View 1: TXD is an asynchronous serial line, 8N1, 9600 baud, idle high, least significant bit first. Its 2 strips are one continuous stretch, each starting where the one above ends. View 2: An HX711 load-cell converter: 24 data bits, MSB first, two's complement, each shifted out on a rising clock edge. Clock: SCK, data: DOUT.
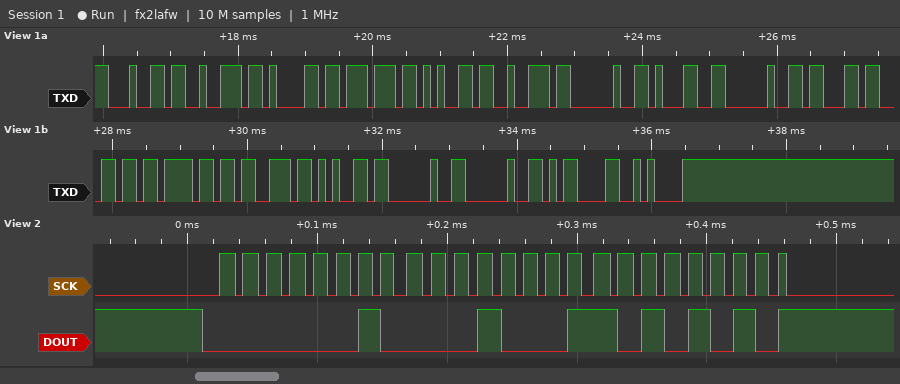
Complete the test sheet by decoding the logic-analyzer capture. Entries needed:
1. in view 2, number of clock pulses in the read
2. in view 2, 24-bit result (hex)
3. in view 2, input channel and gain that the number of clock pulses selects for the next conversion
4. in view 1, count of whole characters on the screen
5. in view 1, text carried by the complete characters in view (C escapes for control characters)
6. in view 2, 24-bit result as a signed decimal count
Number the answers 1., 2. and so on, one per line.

1. 25
2. 0x0211AA
3. channel A, gain 128
4. 18
5. "drawer 1 close  \r\n"
6. 135594
